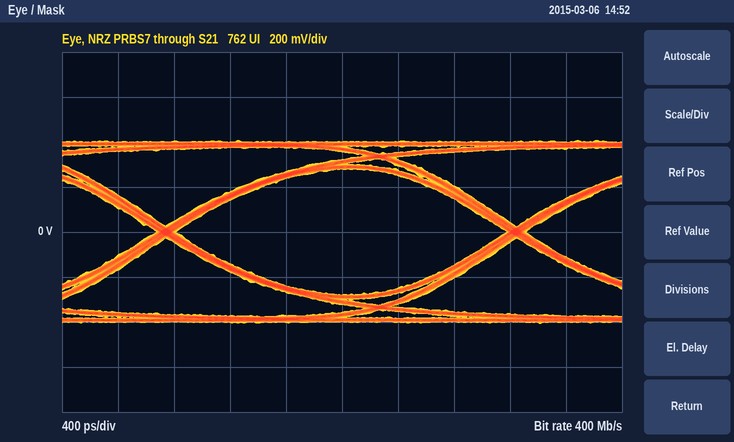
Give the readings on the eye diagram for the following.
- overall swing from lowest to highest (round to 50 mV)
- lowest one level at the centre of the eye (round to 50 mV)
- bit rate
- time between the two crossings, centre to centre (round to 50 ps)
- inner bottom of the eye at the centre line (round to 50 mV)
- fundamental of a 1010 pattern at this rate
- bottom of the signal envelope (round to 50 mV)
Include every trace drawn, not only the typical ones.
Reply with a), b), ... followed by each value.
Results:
a) 800 mV
b) 300 mV
c) 400 Mb/s
d) 2.50 ns
e) -300 mV
f) 200 MHz
g) -400 mV
